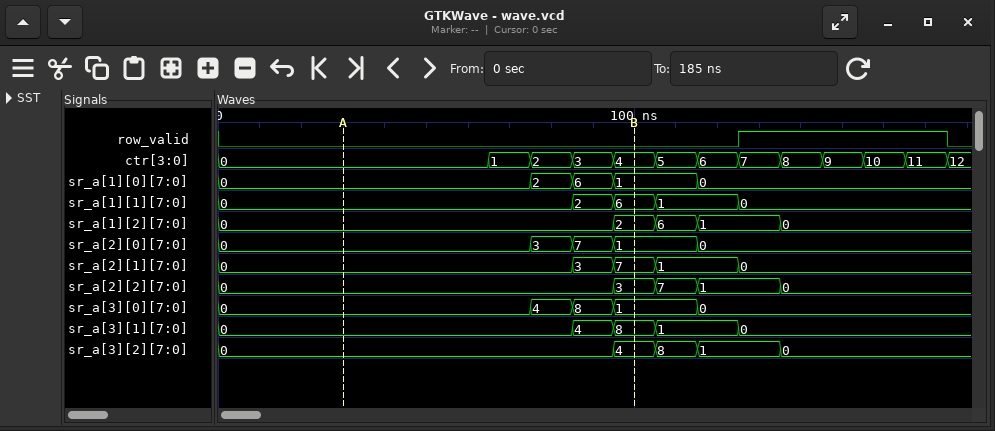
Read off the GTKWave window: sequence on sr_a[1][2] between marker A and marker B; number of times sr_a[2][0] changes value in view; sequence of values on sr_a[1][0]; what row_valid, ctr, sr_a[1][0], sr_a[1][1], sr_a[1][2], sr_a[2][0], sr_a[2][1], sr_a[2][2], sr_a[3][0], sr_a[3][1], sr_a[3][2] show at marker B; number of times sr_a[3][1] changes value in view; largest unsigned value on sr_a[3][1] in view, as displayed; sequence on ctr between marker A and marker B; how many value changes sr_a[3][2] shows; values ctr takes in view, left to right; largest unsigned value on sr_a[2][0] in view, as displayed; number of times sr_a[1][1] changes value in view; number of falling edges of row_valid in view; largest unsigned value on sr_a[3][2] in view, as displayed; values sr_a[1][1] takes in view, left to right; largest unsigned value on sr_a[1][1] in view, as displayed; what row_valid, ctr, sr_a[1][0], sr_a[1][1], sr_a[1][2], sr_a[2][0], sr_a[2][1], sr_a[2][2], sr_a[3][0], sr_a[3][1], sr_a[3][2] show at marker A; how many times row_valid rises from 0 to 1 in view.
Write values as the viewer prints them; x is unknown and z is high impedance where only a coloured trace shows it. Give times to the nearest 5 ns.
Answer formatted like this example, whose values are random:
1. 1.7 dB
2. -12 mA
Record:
1. 0, 2
2. 4
3. 0, 2, 6, 1, 0
4. row_valid=0, ctr=4, sr_a[1][0]=1, sr_a[1][1]=6, sr_a[1][2]=2, sr_a[2][0]=1, sr_a[2][1]=7, sr_a[2][2]=3, sr_a[3][0]=1, sr_a[3][1]=8, sr_a[3][2]=4
5. 4
6. 8
7. 0, 1, 2, 3, 4
8. 4
9. 0, 1, 2, 3, 4, 5, 6, 7, 8, 9, 10, 11, 12
10. 7
11. 4
12. 1
13. 8
14. 0, 2, 6, 1, 0
15. 6
16. row_valid=0, ctr=0, sr_a[1][0]=0, sr_a[1][1]=0, sr_a[1][2]=0, sr_a[2][0]=0, sr_a[2][1]=0, sr_a[2][2]=0, sr_a[3][0]=0, sr_a[3][1]=0, sr_a[3][2]=0
17. 1
